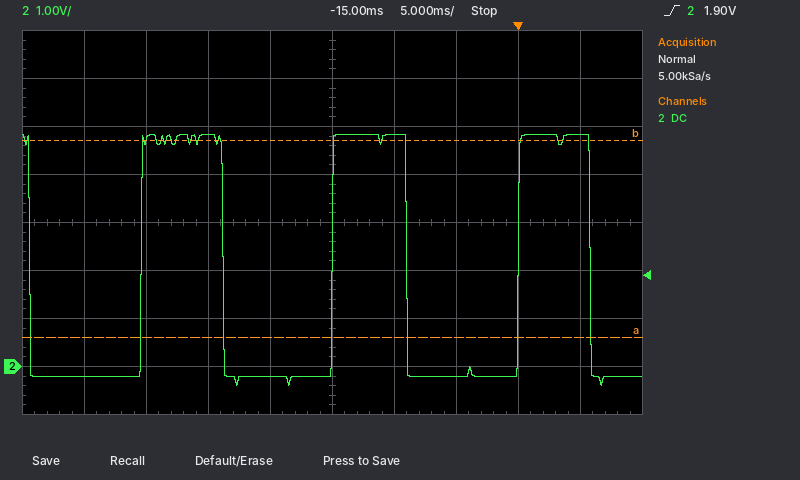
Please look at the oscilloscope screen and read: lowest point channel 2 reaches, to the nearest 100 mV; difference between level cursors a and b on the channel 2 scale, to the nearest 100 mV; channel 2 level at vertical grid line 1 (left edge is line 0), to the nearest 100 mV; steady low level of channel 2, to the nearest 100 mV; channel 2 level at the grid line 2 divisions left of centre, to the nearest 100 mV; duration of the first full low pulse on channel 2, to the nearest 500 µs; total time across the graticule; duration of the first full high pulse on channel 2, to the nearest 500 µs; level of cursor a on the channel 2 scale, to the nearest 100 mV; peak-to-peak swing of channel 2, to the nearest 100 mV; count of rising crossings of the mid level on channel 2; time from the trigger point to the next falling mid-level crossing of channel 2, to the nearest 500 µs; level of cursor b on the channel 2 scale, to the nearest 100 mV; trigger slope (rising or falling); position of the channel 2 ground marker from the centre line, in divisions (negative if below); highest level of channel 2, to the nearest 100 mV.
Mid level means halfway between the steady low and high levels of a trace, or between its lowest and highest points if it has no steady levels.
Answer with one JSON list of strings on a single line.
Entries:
["-400 mV", "4.1 V", "-200 mV", "-200 mV", "4.8 V", "9.0 ms", "50 ms", "6.5 ms", "600 mV", "5.2 V", "3", "6.0 ms", "4.7 V", "rising", "-3.0 div", "4.8 V"]
